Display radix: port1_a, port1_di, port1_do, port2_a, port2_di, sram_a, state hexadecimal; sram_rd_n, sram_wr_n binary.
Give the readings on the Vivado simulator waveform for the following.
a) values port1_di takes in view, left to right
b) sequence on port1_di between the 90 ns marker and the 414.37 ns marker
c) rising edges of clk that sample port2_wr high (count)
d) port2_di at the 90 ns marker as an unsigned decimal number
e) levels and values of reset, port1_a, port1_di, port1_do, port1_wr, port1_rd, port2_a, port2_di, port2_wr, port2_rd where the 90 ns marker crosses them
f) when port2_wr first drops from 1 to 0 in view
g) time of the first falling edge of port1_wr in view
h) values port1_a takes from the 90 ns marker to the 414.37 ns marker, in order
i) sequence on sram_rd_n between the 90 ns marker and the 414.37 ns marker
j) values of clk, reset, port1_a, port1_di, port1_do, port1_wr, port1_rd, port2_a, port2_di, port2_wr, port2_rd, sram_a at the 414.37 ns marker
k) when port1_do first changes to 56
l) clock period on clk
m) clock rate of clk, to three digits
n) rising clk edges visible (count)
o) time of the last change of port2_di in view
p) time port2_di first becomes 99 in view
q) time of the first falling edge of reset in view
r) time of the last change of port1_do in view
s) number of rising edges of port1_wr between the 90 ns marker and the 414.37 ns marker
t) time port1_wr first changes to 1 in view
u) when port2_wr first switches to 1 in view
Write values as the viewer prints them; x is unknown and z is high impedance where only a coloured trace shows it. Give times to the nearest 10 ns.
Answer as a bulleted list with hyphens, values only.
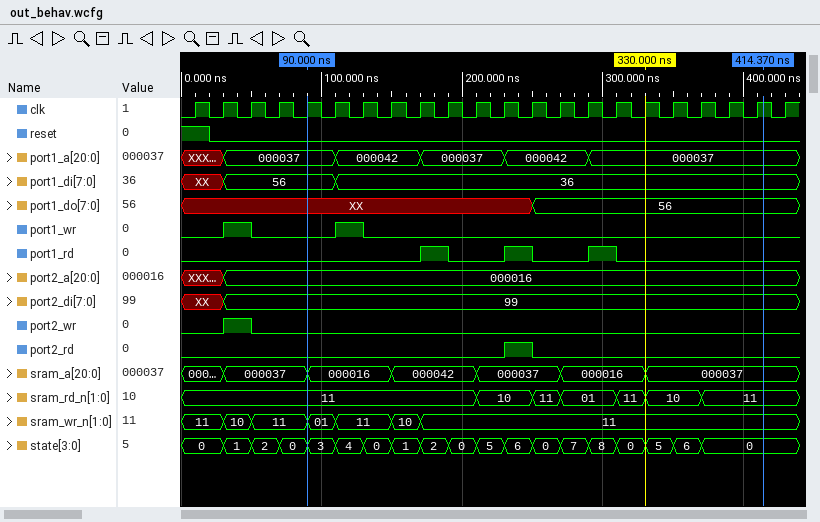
- XX, 56, 36
- 56, 36
- 1
- 153
- reset=0, port1_a=000037, port1_di=56, port1_do=XX, port1_wr=0, port1_rd=0, port2_a=000016, port2_di=99, port2_wr=0, port2_rd=0
- 50 ns
- 50 ns
- 000037, 000042, 000037, 000042, 000037
- 11, 10, 11, 01, 11, 10, 11
- clk=1, reset=0, port1_a=000037, port1_di=36, port1_do=56, port1_wr=0, port1_rd=0, port2_a=000016, port2_di=99, port2_wr=0, port2_rd=0, sram_a=000037
- 250 ns
- 20 ns
- 50.0 MHz
- 22
- 30 ns
- 30 ns
- 20 ns
- 250 ns
- 1
- 30 ns
- 30 ns
